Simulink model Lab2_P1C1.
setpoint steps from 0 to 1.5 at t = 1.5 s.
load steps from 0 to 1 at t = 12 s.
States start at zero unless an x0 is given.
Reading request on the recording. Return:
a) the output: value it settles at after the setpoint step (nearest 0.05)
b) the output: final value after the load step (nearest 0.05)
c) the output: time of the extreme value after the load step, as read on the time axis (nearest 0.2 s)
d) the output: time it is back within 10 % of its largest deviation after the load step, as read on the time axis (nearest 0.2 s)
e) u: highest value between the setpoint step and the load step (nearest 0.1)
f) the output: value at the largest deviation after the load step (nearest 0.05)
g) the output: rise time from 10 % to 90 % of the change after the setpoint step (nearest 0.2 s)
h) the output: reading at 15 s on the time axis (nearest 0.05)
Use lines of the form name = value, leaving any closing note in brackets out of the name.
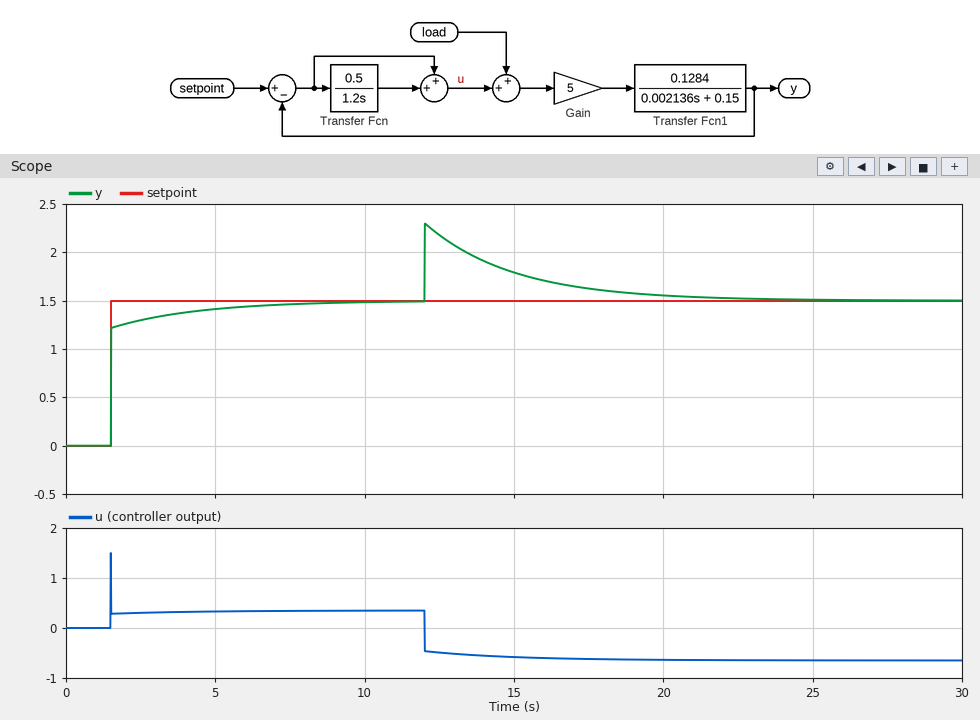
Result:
the output: value it settles at after the setpoint step = 1.50
the output: final value after the load step = 1.50
the output: time of the extreme value after the load step, as read on the time axis = 12.0 s
the output: time it is back within 10 % of its largest deviation after the load step, as read on the time axis = 18.8 s
u: highest value between the setpoint step and the load step = 1.5
the output: value at the largest deviation after the load step = 2.30
the output: rise time from 10 % to 90 % of the change after the setpoint step = 1.8 s
the output: reading at 15 s on the time axis = 1.80
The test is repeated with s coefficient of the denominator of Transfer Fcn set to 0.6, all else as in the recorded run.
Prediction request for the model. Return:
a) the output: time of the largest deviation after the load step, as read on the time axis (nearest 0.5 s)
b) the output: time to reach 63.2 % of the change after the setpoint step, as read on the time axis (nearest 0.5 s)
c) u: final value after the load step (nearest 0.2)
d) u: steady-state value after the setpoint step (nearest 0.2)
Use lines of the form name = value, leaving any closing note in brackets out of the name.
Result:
the output: time of the largest deviation after the load step, as read on the time axis = 12.0 s
the output: time to reach 63.2 % of the change after the setpoint step, as read on the time axis = 1.5 s
u: final value after the load step = -0.6
u: steady-state value after the setpoint step = 0.4
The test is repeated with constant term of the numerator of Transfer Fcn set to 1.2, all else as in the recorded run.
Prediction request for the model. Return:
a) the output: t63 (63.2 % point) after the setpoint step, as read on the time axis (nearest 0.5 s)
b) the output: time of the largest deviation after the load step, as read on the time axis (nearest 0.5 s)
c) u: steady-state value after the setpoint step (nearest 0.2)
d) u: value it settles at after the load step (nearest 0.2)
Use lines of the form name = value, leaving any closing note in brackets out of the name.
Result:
the output: t63 (63.2 % point) after the setpoint step, as read on the time axis = 1.5 s
the output: time of the largest deviation after the load step, as read on the time axis = 12.0 s
u: steady-state value after the setpoint step = 0.4
u: value it settles at after the load step = -0.6
